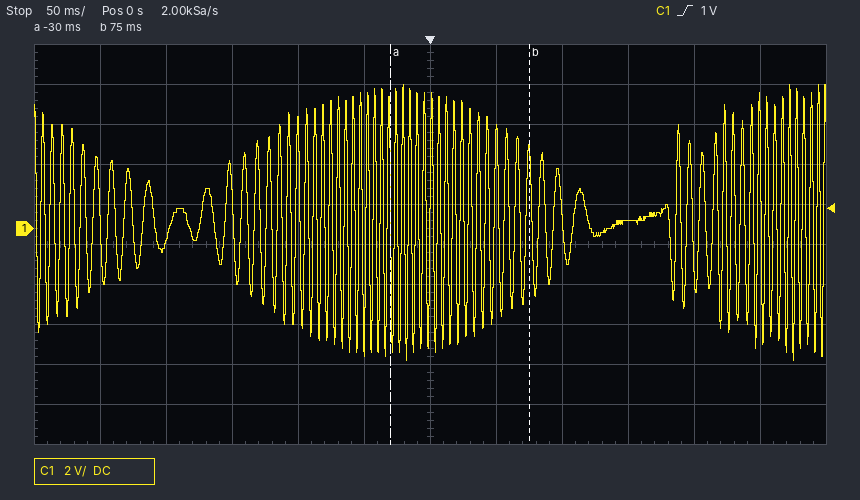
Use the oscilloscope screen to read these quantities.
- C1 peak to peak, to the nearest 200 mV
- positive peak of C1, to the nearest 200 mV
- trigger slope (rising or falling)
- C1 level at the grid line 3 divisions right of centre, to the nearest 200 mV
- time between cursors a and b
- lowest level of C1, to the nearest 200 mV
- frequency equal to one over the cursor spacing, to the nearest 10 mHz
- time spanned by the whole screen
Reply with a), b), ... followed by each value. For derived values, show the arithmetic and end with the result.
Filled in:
a) 7.2 V − (-6.6 V) = 13.8 V
b) 7.2 V
c) rising
d) 400 mV
e) 75 ms − (-30 ms) = 105 ms
f) -6.6 V
g) 1 / 105 ms ≈ 9.52 Hz
h) 600 ms
